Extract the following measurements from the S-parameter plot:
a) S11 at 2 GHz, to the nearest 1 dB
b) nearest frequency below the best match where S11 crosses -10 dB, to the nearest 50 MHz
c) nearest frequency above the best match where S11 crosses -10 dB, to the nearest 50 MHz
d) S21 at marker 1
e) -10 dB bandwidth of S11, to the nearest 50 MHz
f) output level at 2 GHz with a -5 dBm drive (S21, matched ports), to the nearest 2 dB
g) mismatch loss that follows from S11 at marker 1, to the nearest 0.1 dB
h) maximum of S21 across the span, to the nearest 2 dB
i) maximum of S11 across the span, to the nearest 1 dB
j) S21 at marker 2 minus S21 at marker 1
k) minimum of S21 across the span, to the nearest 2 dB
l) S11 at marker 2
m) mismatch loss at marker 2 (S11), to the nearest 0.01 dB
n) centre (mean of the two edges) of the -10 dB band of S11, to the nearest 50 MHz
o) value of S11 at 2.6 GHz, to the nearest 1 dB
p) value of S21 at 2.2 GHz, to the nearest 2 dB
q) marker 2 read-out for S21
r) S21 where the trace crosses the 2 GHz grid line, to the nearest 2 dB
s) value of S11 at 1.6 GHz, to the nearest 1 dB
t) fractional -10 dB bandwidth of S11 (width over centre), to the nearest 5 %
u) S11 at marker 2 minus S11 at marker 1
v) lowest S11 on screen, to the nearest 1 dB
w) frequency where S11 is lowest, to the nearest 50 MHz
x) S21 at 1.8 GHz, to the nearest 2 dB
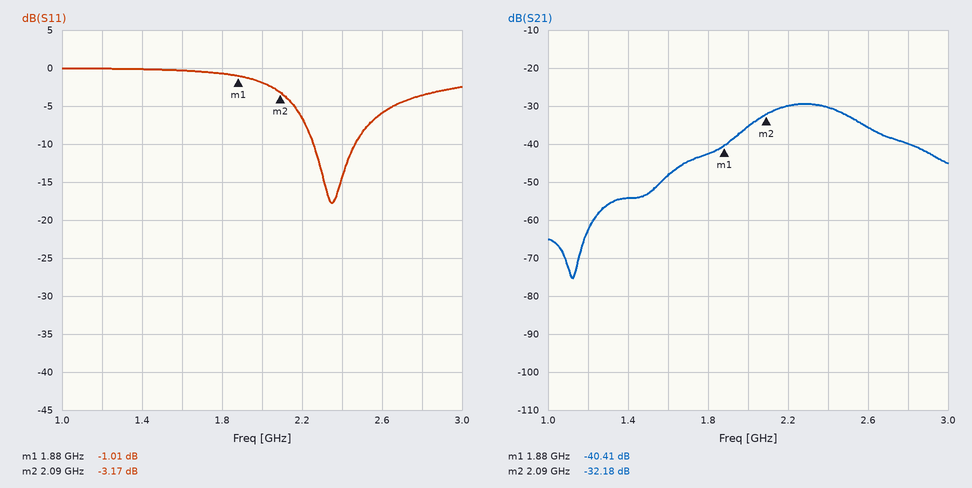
-2 dB
2.25 GHz
2.45 GHz
-40.41 dB
200 MHz
-40 dBm
6.8 dB
-30 dB
0 dB
8.23 dB
-76 dB
-3.17 dB
2.86 dB
2.35 GHz
-6 dB
-30 dB
-32.18 dB
-36 dB
0 dB
10 %
-2.16 dB
-18 dB
2.35 GHz
-42 dB
